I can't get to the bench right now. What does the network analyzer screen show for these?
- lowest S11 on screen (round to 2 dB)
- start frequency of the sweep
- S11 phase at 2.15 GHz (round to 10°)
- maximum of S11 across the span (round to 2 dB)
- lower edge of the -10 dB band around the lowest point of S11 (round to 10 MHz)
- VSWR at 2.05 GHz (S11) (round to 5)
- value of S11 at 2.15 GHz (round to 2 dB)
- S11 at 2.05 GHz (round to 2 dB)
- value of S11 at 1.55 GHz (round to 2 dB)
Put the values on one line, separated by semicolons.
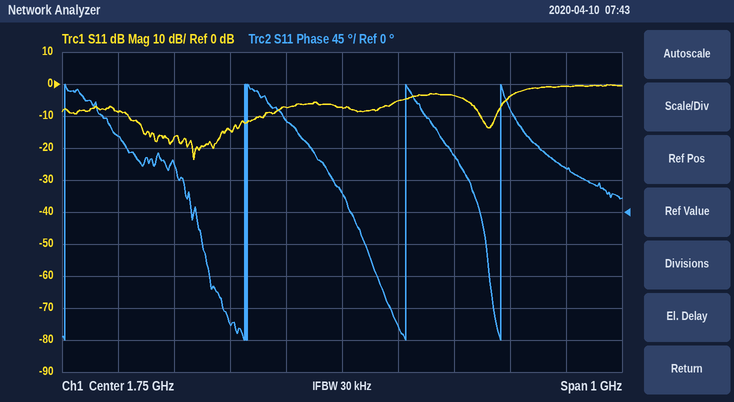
-24 dB; 1.25 GHz; 60°; 0 dB; 1.37 GHz; 5; 0 dB; -4 dB; -14 dB
